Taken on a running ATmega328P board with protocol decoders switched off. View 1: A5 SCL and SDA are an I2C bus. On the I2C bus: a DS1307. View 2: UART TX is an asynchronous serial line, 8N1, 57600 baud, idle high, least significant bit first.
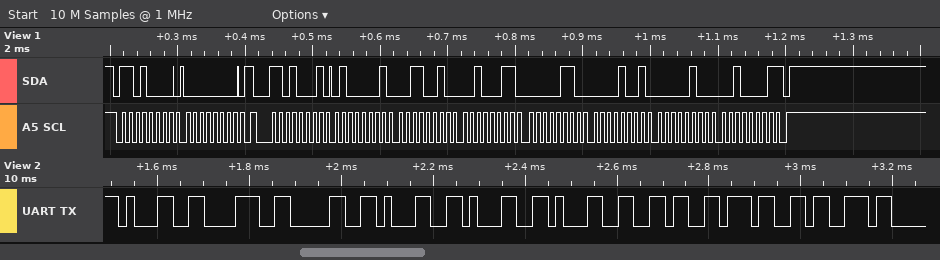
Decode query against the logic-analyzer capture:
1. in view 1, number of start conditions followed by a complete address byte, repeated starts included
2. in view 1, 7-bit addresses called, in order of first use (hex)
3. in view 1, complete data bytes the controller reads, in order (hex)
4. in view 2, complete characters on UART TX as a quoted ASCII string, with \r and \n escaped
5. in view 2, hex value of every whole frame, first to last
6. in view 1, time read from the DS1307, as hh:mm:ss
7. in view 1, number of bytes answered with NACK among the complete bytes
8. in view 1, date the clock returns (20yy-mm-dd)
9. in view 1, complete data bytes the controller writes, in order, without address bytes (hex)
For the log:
2
0x68
41 32 23 06 09 04 21
"18011167s"
31 38 30 31 31 31 36 37 73
23:32:41
1
2021-04-09
00
